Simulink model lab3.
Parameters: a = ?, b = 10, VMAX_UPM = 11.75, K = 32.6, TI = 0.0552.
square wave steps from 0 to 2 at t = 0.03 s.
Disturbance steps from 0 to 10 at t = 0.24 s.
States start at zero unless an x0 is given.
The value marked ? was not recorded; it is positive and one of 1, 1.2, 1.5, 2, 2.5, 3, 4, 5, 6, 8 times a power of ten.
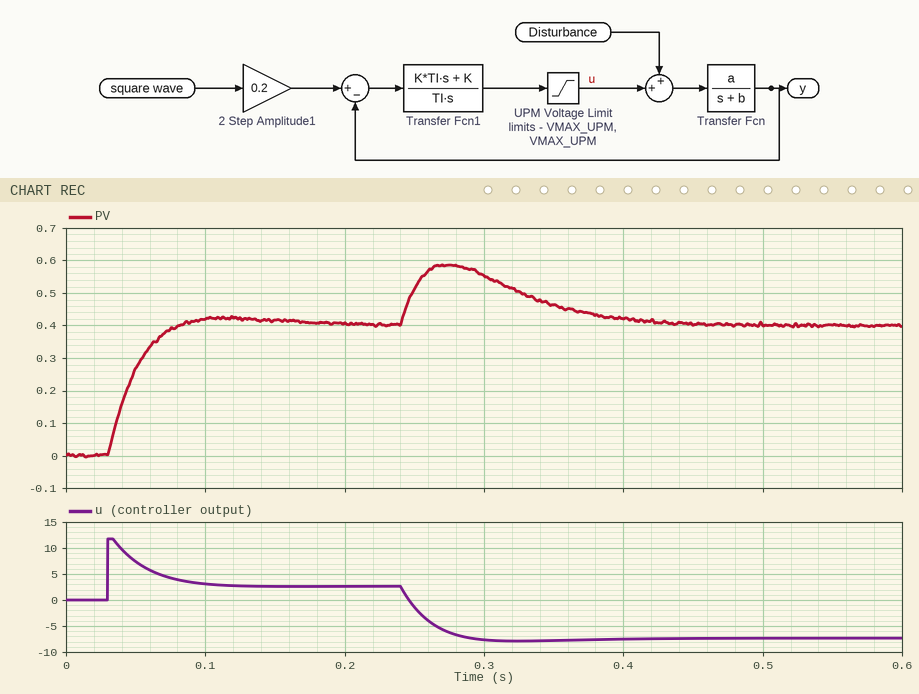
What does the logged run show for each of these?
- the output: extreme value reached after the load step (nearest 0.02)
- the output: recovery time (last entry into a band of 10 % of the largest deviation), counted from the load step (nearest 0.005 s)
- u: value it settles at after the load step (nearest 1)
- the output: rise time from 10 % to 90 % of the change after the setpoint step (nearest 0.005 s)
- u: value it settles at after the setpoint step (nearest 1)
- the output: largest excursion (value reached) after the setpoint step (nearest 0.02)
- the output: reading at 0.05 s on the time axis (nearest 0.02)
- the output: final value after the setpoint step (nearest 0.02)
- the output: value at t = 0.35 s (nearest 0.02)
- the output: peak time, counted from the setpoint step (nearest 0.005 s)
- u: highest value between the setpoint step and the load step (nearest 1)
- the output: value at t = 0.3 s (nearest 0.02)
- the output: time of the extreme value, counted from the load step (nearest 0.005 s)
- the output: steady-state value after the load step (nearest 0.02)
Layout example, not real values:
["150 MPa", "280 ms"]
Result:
["0.58", "0.165 s", "-7", "0.035 s", "3", "0.42", "0.26", "0.40", "0.46", "0.085 s", "12", "0.56", "0.035 s", "0.40"]
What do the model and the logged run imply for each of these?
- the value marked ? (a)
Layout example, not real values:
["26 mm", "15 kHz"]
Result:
["1.5"]
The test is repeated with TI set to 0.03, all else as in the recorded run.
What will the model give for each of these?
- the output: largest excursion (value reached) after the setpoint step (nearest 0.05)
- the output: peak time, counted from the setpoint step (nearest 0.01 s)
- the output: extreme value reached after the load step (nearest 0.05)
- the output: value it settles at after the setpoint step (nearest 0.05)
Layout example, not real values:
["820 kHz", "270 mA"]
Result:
["0.45", "0.06 s", "0.55", "0.40"]
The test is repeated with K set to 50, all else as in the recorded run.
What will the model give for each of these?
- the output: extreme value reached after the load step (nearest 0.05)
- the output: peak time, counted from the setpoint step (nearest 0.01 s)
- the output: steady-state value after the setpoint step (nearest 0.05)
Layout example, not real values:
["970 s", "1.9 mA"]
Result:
["0.55", "0.06 s", "0.40"]
